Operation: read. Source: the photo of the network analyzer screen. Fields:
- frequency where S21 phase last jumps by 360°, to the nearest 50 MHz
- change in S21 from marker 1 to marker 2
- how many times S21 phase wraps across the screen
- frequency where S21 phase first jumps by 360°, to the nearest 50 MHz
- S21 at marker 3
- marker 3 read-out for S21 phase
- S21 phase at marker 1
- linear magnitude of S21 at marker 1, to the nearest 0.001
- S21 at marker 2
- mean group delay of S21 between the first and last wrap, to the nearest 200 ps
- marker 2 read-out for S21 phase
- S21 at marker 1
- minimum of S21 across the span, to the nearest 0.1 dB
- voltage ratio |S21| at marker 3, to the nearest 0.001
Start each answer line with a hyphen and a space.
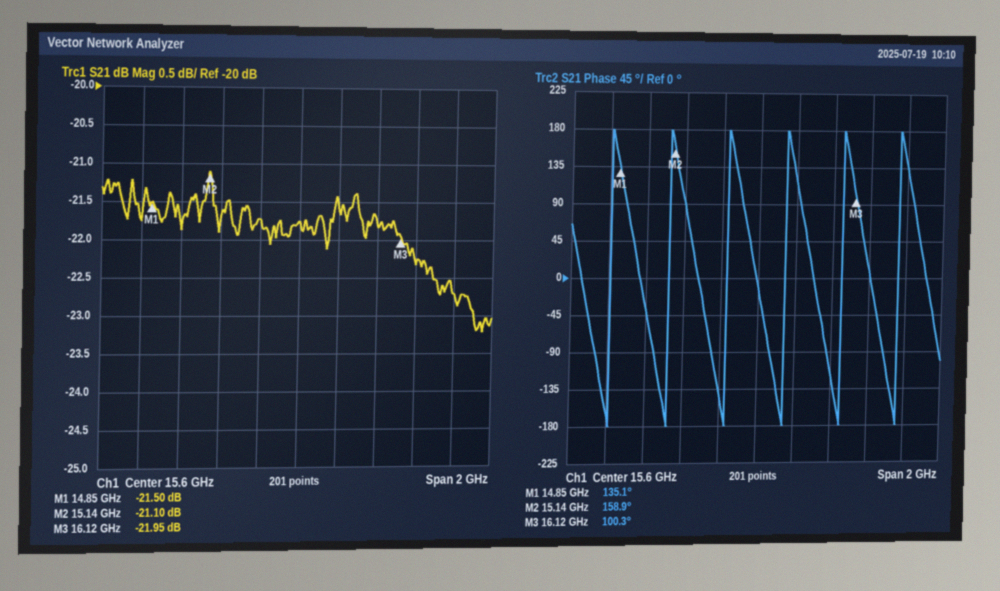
- 16.35 GHz
- 0.40 dB
- 6
- 14.80 GHz
- -21.95 dB
- 100.3°
- 135.1°
- 0.084
- -21.10 dB
- 3.2 ns
- 158.9°
- -21.50 dB
- -23.2 dB
- 0.080
